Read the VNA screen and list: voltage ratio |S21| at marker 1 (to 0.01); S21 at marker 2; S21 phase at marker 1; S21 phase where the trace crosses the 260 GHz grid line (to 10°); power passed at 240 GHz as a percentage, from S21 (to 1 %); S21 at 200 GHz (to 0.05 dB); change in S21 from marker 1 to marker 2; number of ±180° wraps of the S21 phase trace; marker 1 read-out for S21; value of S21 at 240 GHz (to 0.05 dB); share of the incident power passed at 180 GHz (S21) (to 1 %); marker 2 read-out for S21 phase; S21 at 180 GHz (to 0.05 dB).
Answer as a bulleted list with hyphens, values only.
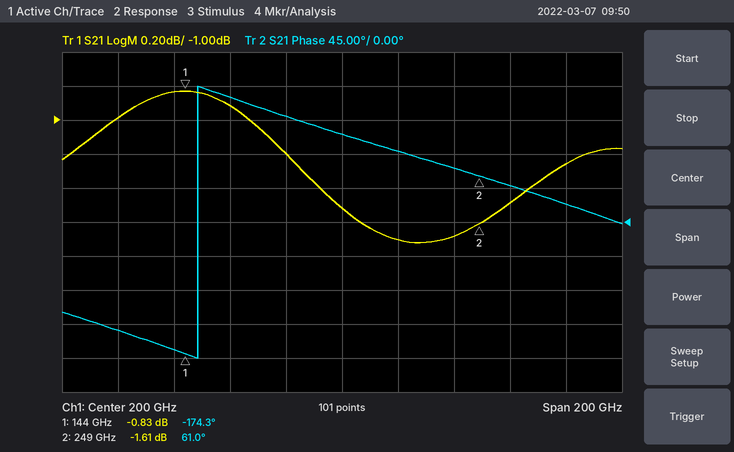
- 0.91
- -1.61 dB
- -174.3°
- 50°
- 68 %
- -1.50 dB
- -0.78 dB
- 1
- -0.83 dB
- -1.70 dB
- 76 %
- 61.0°
- -1.20 dB
